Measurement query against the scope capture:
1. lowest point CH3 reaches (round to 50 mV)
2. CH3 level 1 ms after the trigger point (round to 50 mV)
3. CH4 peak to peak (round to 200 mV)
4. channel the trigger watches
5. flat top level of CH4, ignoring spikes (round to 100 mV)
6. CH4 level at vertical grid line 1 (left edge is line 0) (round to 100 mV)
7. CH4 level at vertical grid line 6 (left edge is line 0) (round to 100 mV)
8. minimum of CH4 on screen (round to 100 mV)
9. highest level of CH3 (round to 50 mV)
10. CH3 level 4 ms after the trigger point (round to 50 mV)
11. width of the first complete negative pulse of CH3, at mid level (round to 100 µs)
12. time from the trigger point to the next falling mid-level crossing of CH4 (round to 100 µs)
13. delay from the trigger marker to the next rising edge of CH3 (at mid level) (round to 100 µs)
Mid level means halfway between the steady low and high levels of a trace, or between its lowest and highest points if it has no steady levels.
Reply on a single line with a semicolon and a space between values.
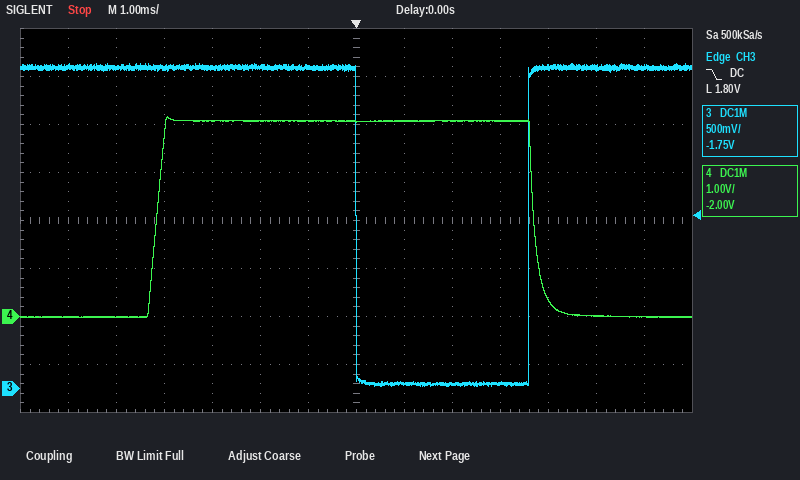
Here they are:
0 mV; 50 mV; 4.2 V; CH3; 4.1 V; 0.0 V; 4.1 V; 0.0 V; 3.40 V; 3.35 V; 3.6 ms; 3.7 ms; 3.6 ms
